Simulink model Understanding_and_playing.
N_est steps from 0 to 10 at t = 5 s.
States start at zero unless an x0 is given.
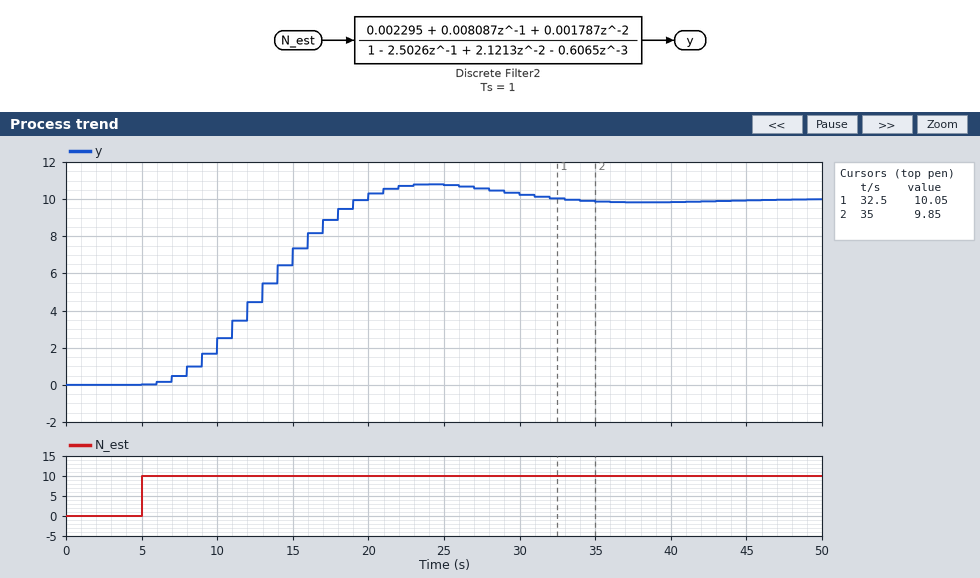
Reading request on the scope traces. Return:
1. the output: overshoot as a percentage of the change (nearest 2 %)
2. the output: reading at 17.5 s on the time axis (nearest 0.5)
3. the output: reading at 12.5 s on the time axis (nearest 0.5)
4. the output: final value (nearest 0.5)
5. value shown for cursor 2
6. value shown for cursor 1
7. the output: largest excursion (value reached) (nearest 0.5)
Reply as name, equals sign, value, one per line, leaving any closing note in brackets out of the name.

the output: overshoot as a percentage of the change = 8 %
the output: reading at 17.5 s on the time axis = 9.0
the output: reading at 12.5 s on the time axis = 4.5
the output: final value = 10.0
value shown for cursor 2 = 9.85
value shown for cursor 1 = 10.05
the output: largest excursion (value reached) = 11.0
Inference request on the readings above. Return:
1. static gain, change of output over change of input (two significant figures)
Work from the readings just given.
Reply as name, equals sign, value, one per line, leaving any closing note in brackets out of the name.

static gain, change of output over change of input = 1.0
